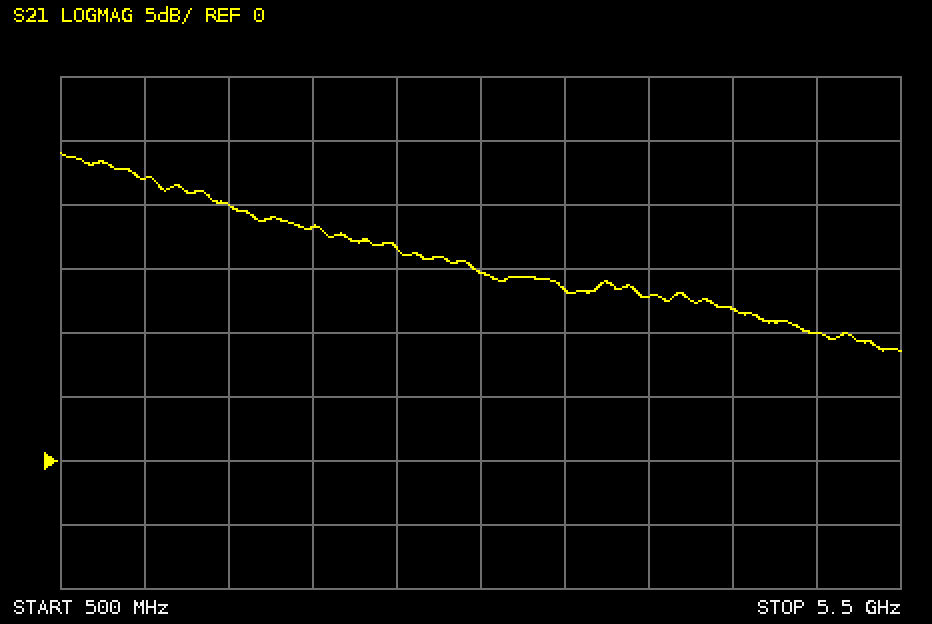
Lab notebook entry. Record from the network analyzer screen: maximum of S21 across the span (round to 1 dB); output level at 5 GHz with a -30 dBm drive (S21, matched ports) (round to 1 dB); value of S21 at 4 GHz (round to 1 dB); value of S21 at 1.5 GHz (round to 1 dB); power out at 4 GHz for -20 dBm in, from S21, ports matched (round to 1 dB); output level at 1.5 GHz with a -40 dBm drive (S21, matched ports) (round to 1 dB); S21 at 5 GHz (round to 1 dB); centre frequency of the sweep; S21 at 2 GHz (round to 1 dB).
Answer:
24 dB
-20 dBm
13 dB
20 dB
-7 dBm
-20 dBm
10 dB
3 GHz
18 dB
